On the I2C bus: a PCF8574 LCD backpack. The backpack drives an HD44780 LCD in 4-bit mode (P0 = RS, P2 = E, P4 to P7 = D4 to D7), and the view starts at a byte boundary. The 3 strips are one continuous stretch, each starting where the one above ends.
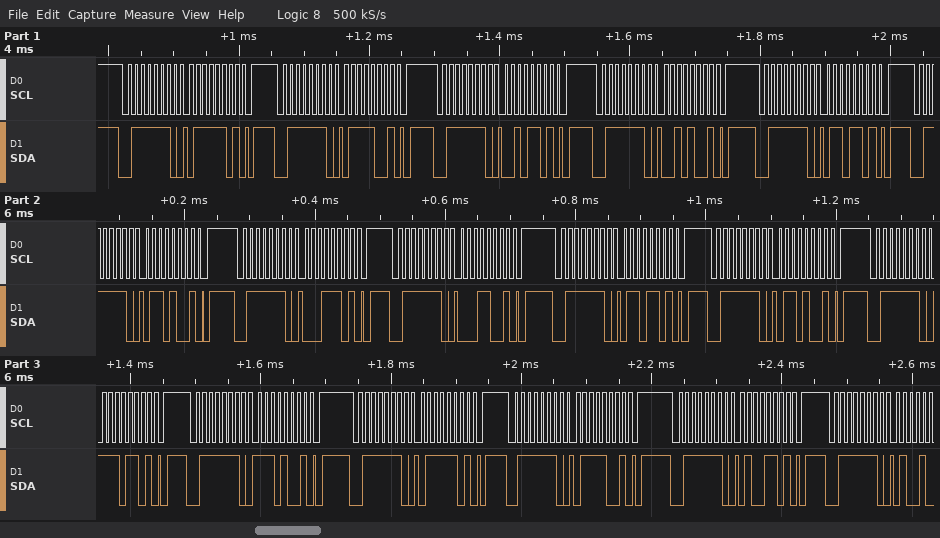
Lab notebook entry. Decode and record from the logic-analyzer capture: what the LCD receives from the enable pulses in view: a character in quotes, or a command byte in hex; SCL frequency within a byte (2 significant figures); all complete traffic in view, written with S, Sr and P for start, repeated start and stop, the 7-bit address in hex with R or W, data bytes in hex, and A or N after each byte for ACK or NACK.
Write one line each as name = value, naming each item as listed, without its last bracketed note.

what the LCD receives from the enable pulses in view: a character in quotes, or a command byte in hex = 'r' 'a' 'n'
SCL frequency within a byte = 100 kHz
all complete traffic in view, written with S, Sr and P for start, repeated start and stop, the 7-bit address in hex with R or W, data bytes in hex, and A or N after each byte for ACK or NACK = S 3FW A 7D A P S 3FW A 79 A P S 3FW A 2D A P S 3FW A 29 A P S 3FW A 6D A P S 3FW A 69 A P S 3FW A 1D A P S 3FW A 19 A P S 3FW A 6D A P S 3FW A 69 A P S 3FW A ED A P S 3FW A E9 A P S 3FW A 7D A P S 3FW A 79 A P S 3FW A 4D A P S 3FW A
